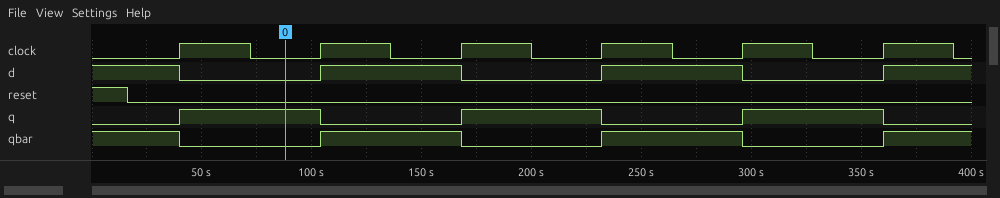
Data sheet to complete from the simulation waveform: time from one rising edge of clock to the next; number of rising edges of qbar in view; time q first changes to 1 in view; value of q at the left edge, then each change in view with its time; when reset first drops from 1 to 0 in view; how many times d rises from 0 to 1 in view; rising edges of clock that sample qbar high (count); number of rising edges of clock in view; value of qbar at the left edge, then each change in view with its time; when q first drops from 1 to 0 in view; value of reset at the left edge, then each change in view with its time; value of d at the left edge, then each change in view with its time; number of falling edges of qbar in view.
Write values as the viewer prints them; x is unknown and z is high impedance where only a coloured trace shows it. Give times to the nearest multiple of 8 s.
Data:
64 s
3
40 s
0, 1 at 40 s, 0 at 104 s, 1 at 168 s, 0 at 232 s, 1 at 296 s, 0 at 360 s
16 s
3
3
6
1, 0 at 40 s, 1 at 104 s, 0 at 168 s, 1 at 232 s, 0 at 296 s, 1 at 360 s
104 s
1, 0 at 16 s
1, 0 at 40 s, 1 at 104 s, 0 at 168 s, 1 at 232 s, 0 at 296 s, 1 at 360 s
3
